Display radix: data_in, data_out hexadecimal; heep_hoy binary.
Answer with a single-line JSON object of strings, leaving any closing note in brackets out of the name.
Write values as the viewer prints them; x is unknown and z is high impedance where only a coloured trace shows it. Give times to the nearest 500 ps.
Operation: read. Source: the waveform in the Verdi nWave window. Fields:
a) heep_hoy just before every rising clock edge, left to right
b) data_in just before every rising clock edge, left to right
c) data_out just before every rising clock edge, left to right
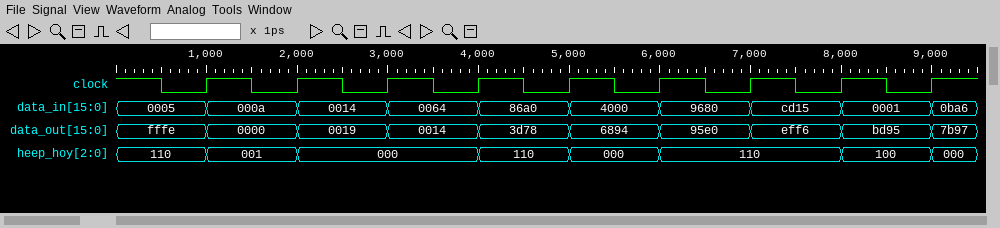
{"heep_hoy just before every rising clock edge, left to right": "110, 001, 000, 000, 110, 000, 110, 110, 100", "data_in just before every rising clock edge, left to right": "0005, 000a, 0014, 0064, 86a0, 4000, 9680, cd15, 0001", "data_out just before every rising clock edge, left to right": "fffe, 0000, 0019, 0014, 3d78, 6894, 95e0, eff6, bd95"}
